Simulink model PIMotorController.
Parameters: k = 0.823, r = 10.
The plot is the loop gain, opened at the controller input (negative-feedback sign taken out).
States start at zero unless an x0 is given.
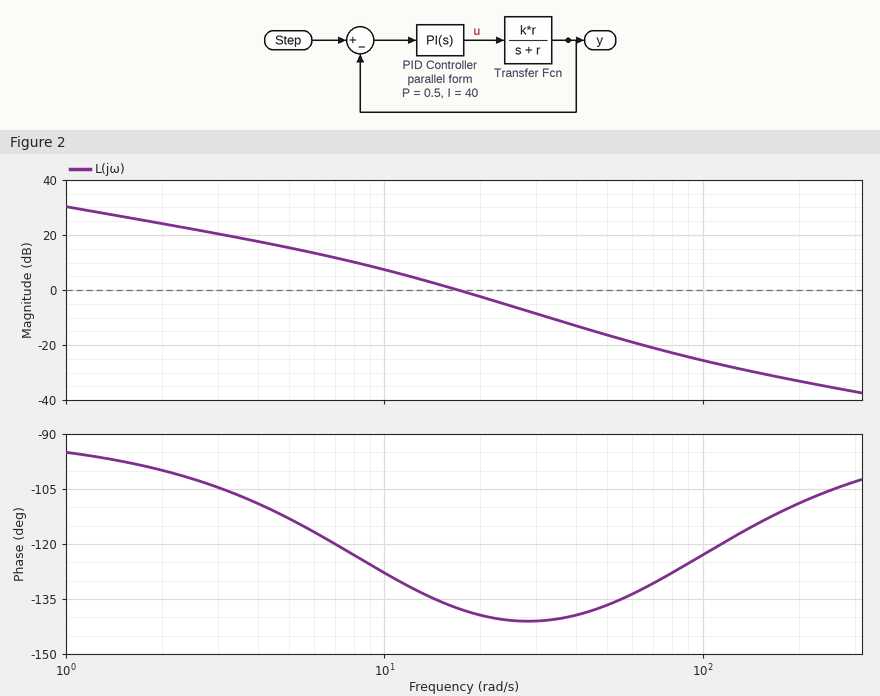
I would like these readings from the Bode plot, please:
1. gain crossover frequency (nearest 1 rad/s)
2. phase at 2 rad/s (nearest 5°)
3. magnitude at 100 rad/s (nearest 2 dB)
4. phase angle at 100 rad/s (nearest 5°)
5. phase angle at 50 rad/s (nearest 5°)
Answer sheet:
17 rad/s
-100°
-26 dB
-125°
-135°
